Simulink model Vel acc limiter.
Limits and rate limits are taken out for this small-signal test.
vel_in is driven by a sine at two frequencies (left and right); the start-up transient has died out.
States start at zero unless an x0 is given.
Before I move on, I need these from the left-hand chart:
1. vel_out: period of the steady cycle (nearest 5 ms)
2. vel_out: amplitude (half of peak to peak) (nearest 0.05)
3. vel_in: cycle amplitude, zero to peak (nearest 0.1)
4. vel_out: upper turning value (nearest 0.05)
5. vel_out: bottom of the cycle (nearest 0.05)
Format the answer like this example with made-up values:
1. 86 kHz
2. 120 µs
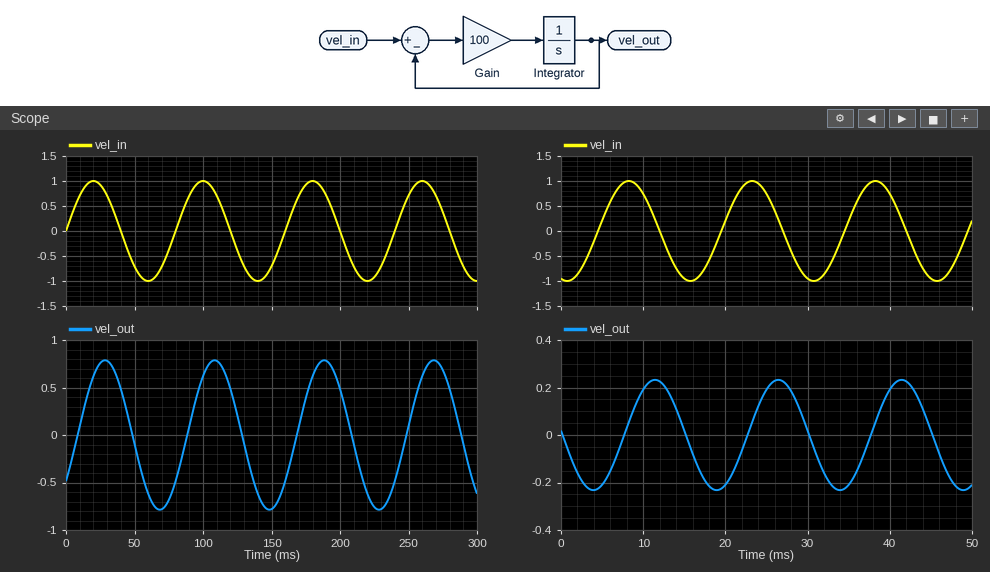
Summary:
1. 80 ms
2. 0.80
3. 1.0
4. 0.80
5. -0.80
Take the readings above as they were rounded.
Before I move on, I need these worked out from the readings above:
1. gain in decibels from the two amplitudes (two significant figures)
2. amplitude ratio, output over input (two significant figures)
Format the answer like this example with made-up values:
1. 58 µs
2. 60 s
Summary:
1. -1.9 dB
2. 0.80
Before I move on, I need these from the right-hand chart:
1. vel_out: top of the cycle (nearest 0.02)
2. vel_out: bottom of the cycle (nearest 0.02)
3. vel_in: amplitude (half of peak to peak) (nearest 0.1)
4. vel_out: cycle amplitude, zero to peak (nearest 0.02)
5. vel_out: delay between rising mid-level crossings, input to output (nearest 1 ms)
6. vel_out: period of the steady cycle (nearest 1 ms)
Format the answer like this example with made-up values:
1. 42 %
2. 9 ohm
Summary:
1. 0.24
2. -0.24
3. 1.0
4. 0.24
5. 3 ms
6. 15 ms
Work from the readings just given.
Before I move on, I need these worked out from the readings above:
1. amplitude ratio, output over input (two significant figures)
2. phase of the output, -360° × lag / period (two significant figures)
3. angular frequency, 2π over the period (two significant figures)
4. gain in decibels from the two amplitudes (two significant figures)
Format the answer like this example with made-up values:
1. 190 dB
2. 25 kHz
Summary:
1. 0.24
2. -72°
3. 0.42 rad/ms
4. -12 dB
